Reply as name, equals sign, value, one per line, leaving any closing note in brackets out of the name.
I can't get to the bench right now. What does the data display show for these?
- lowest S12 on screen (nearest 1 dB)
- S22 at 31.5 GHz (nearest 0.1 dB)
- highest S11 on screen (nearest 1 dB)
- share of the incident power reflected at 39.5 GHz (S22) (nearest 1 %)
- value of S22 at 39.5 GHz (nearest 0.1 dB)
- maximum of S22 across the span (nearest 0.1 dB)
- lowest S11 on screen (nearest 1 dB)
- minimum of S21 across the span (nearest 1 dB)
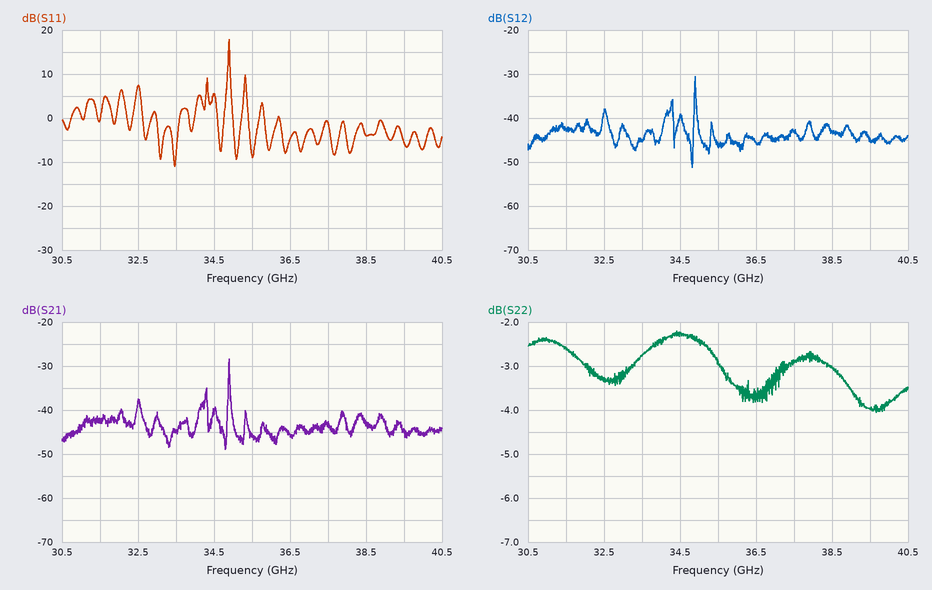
lowest S12 on screen = -51 dB
S22 at 31.5 GHz = -2.6 dB
highest S11 on screen = 18 dB
share of the incident power reflected at 39.5 GHz (S22) = 40 %
value of S22 at 39.5 GHz = -4.0 dB
maximum of S22 across the span = -2.2 dB
lowest S11 on screen = -11 dB
minimum of S21 across the span = -49 dB
